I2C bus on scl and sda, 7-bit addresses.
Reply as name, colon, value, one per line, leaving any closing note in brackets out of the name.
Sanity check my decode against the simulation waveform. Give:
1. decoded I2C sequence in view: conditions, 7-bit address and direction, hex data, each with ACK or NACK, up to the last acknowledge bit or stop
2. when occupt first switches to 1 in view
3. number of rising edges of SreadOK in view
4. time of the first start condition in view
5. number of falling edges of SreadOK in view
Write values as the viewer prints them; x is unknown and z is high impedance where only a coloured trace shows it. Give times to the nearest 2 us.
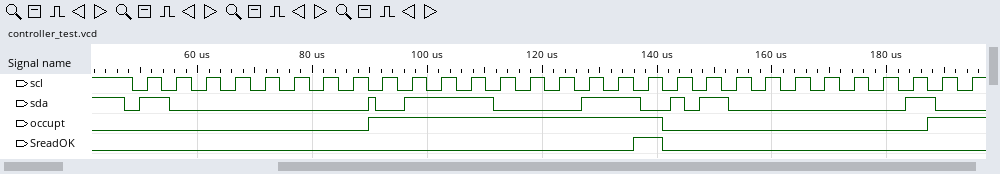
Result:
decoded I2C sequence in view: conditions, 7-bit address and direction, hex data, each with ACK or NACK, up to the last acknowledge bit or stop: start, address 40 write ACK, E3 ACK, repeated start, address 40 read ACK
when occupt first switches to 1 in view: 90 us
number of rising edges of SreadOK in view: 1
time of the first start condition in view: 48 us
number of falling edges of SreadOK in view: 1
